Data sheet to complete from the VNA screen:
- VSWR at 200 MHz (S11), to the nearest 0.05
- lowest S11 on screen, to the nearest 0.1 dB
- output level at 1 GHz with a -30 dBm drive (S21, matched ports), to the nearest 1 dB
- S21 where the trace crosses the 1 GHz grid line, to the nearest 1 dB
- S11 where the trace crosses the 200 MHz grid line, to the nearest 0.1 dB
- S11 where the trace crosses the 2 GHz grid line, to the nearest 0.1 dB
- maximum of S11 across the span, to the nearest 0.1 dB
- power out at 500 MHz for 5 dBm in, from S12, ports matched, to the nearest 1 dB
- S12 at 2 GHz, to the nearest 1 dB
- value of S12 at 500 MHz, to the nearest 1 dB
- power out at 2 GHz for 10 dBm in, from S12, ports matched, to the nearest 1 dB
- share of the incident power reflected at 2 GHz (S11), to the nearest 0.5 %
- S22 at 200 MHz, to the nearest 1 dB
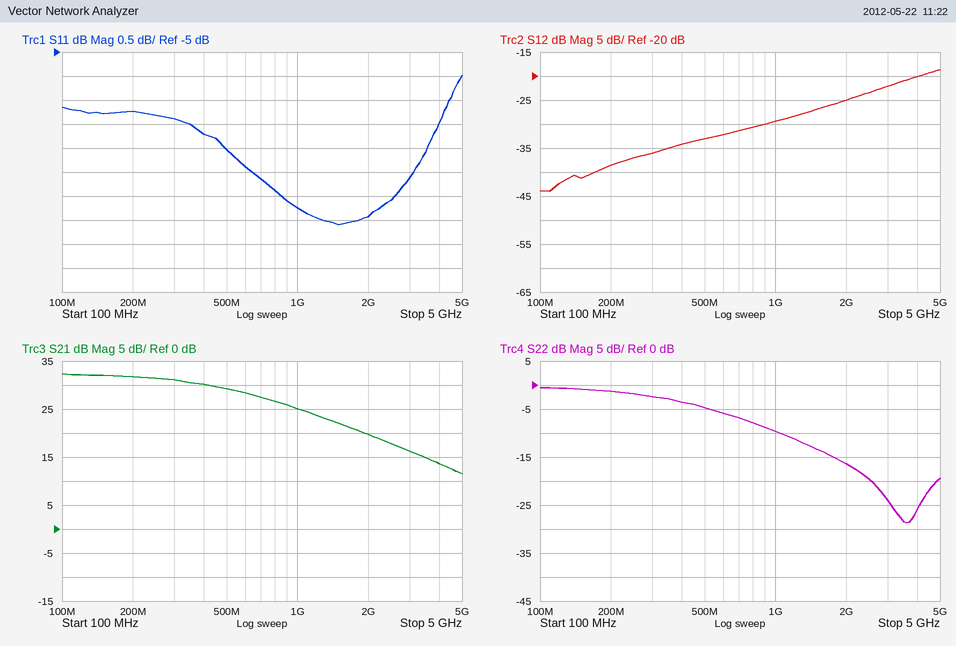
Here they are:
2.90
-8.6 dB
-5 dBm
25 dB
-6.2 dB
-8.4 dB
-5.5 dB
-28 dBm
-25 dB
-33 dB
-15 dBm
14.5 %
-1 dB
